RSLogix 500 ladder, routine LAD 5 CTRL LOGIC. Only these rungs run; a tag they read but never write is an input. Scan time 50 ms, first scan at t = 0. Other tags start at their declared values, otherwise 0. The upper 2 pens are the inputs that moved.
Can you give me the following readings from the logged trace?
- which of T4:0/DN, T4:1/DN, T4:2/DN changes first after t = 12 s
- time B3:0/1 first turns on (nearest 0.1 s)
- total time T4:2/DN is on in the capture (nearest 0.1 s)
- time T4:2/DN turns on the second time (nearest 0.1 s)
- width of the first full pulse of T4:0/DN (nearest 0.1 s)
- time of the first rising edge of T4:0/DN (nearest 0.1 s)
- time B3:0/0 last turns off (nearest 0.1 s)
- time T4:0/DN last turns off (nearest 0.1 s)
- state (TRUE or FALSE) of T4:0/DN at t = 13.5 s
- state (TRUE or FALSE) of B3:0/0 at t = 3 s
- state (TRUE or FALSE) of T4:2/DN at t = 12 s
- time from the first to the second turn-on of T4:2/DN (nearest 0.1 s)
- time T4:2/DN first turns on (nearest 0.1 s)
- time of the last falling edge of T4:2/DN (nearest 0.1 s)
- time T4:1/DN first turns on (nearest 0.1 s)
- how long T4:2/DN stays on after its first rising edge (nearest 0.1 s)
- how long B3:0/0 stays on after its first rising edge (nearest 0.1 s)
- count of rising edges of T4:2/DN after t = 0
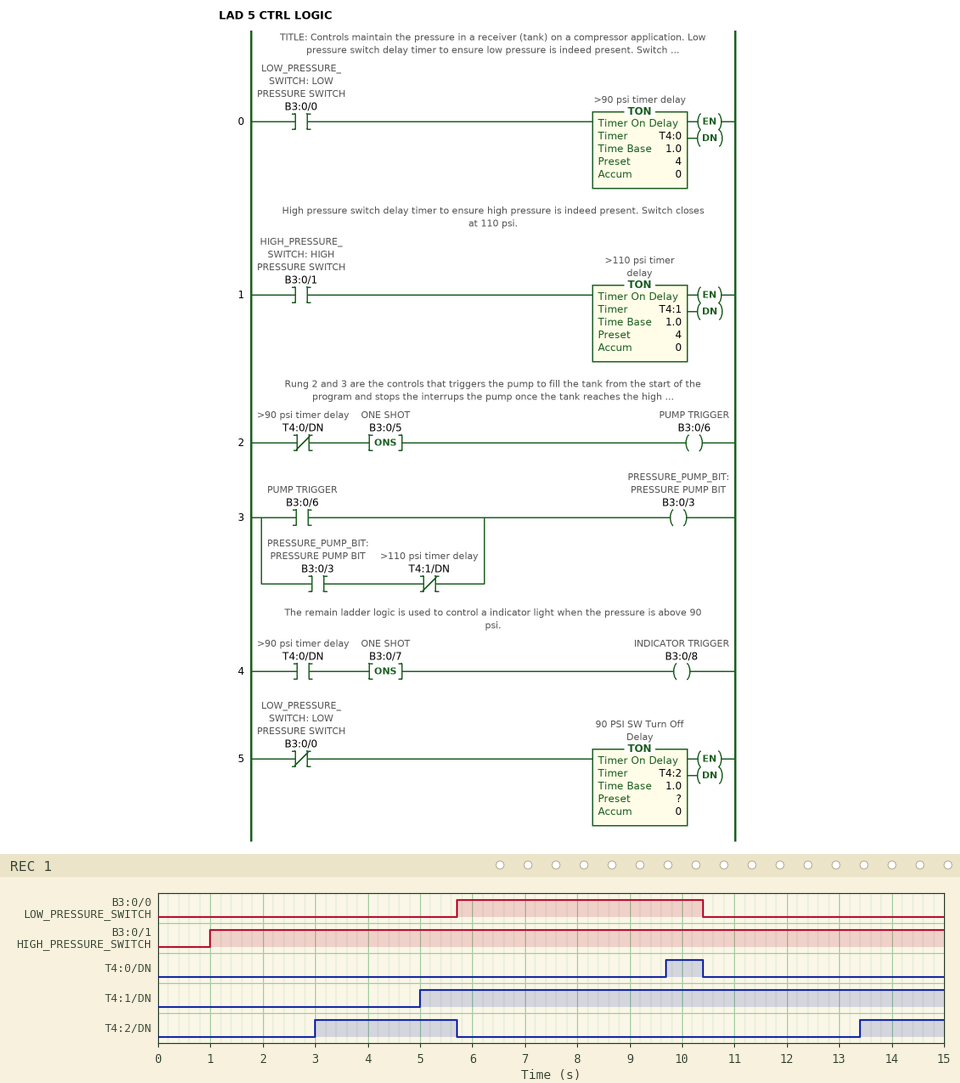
T4:2/DN
1.0 s
4.3 s
13.4 s
0.7 s
9.7 s
10.4 s
10.4 s
FALSE
FALSE
FALSE
10.4 s
3.0 s
5.7 s
5.0 s
2.7 s
4.7 s
2
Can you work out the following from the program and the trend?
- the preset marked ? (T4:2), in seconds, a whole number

3 s
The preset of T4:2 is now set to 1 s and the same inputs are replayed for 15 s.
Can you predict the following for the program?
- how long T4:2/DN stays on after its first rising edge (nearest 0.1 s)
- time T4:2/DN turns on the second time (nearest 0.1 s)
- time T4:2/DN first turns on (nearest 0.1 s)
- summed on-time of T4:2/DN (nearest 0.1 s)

4.7 s
11.4 s
1.0 s
8.3 s
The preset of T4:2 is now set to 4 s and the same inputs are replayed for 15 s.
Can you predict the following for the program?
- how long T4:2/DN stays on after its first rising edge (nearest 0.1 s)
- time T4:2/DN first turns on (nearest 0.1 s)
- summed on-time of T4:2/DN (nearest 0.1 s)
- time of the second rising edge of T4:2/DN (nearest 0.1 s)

1.7 s
4.0 s
2.3 s
14.4 s
